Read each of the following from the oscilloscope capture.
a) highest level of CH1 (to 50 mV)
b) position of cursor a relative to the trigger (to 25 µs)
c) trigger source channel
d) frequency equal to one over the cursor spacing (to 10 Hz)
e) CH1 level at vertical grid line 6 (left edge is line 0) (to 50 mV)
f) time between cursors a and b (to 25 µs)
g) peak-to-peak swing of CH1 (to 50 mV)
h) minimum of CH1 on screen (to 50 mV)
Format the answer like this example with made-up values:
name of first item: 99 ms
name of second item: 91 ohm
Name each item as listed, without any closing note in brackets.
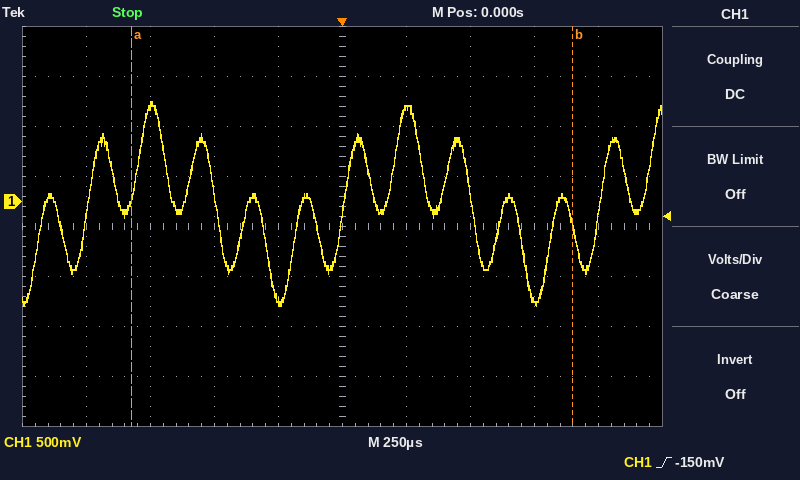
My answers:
highest level of CH1: 1.00 V
position of cursor a relative to the trigger: -825 µs
trigger source channel: CH1
frequency equal to one over the cursor spacing: 580 Hz
CH1 level at vertical grid line 6 (left edge is line 0): 900 mV
time between cursors a and b: 1.725 ms
peak-to-peak swing of CH1: 2.05 V
minimum of CH1 on screen: -1.05 V
